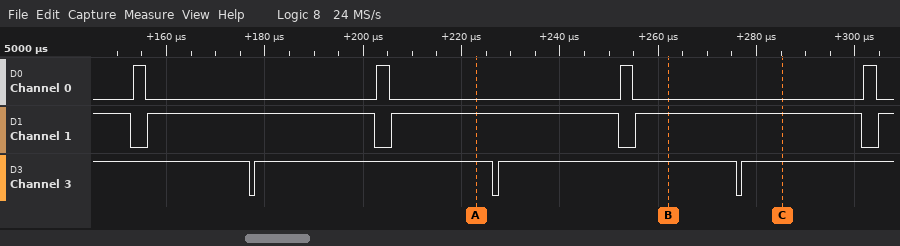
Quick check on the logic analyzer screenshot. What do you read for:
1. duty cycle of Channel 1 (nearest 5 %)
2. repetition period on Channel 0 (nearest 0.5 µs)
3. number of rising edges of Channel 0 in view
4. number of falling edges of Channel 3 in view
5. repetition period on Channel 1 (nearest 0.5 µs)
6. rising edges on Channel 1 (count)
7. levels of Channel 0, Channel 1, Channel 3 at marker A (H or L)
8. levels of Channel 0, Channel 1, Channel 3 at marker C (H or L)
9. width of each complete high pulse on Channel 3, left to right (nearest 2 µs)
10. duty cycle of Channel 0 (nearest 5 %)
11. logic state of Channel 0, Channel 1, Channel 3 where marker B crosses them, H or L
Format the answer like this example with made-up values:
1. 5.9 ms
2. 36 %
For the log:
1. 95 %
2. 49.5 µs
3. 4
4. 3
5. 49.5 µs
6. 4
7. Channel 0=L, Channel 1=H, Channel 3=H
8. Channel 0=L, Channel 1=H, Channel 3=H
9. 48 µs, 48 µs
10. 5 %
11. Channel 0=L, Channel 1=H, Channel 3=H
